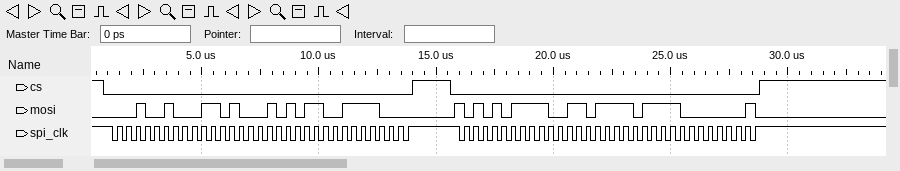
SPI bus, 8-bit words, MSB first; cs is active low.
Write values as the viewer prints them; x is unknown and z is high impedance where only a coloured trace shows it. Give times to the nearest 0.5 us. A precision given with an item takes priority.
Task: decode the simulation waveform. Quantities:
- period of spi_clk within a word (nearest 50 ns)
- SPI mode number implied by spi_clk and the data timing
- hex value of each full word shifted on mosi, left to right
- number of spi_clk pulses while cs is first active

400 ns
2
12, 34, 56, 78, AB, CD, EF, 01
32
